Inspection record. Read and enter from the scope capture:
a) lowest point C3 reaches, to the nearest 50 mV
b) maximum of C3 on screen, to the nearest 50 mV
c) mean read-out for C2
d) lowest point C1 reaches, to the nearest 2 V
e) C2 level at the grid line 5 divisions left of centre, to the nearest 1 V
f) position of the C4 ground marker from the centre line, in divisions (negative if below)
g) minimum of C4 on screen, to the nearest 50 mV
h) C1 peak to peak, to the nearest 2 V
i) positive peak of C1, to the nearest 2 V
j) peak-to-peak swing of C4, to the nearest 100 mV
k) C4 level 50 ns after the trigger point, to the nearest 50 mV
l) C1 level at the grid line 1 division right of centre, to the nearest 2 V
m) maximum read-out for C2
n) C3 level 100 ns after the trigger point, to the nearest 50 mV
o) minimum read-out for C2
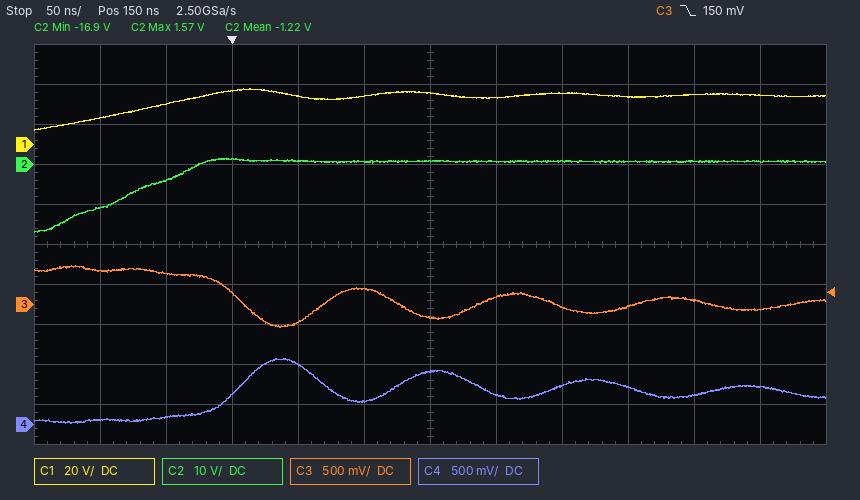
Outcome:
-300 mV
500 mV
-1.22 V
8 V
-11 V
-4.5 div
0 mV
20 V
28 V
800 mV
750 mV
24 V
1.57 V
200 mV
-16.9 V
